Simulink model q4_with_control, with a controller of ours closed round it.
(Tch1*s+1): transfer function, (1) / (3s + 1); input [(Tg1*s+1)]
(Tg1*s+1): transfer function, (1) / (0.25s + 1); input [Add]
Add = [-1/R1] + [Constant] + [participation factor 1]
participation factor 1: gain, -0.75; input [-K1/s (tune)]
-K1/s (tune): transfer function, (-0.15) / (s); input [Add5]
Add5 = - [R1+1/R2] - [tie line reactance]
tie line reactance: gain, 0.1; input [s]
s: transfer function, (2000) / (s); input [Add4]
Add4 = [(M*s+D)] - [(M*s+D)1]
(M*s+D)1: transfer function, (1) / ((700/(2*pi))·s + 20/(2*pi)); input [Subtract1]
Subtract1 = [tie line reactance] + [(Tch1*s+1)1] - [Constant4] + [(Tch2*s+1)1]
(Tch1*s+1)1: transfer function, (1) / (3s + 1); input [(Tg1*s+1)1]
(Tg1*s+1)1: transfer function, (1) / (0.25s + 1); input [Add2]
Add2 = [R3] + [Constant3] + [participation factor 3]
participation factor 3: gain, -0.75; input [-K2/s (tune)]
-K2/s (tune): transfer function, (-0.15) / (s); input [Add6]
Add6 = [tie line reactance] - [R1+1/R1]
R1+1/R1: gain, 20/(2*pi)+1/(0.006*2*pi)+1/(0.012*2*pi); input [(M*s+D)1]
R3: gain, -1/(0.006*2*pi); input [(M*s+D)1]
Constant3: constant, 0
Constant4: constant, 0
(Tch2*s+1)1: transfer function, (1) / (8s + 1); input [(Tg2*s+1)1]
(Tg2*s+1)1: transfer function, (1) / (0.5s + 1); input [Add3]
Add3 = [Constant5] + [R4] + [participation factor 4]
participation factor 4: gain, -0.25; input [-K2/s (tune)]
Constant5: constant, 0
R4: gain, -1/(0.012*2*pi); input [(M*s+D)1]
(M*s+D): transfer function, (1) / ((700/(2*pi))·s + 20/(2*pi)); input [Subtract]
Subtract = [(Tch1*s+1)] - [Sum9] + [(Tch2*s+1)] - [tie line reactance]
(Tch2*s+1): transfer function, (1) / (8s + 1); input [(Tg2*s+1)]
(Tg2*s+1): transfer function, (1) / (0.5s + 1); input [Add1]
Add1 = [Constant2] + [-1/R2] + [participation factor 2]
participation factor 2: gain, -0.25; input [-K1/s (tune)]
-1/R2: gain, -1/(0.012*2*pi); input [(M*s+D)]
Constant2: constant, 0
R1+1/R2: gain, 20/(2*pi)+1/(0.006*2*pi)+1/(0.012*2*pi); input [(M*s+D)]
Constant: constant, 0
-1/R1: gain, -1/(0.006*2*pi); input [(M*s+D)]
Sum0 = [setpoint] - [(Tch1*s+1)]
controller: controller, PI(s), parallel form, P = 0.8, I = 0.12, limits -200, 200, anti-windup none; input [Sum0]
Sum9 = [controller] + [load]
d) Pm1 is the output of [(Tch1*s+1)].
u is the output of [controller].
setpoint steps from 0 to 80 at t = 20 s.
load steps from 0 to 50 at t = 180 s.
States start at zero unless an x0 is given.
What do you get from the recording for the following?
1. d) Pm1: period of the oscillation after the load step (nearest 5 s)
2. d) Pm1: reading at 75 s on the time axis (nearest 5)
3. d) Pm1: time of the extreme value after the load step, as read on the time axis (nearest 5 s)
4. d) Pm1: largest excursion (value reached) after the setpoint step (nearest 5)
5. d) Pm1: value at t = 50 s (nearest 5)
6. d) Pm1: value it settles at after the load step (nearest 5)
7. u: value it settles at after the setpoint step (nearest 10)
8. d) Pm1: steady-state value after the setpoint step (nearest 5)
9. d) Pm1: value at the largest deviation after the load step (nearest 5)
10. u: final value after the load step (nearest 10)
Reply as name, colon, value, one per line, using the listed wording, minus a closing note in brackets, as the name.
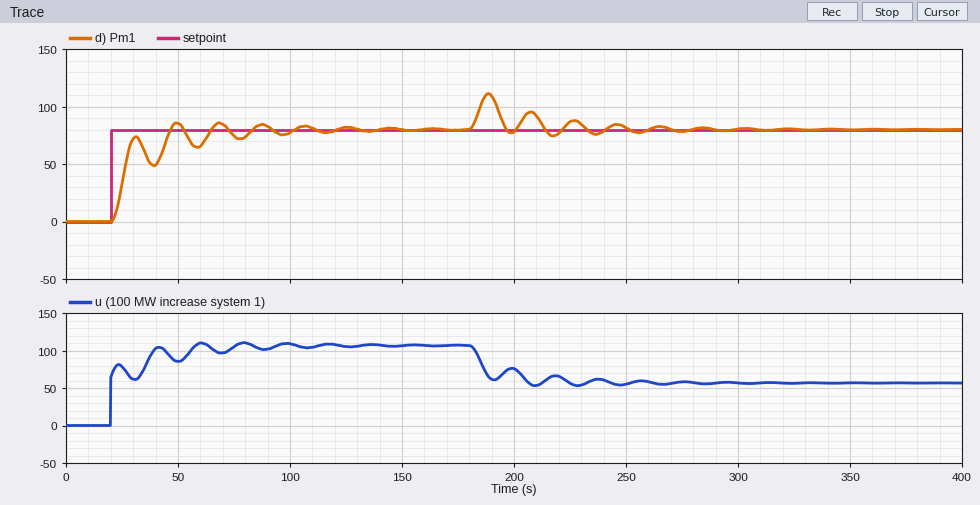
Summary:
d) Pm1: period of the oscillation after the load step: 20 s
d) Pm1: reading at 75 s on the time axis: 75
d) Pm1: time of the extreme value after the load step, as read on the time axis: 190 s
d) Pm1: largest excursion (value reached) after the setpoint step: 85
d) Pm1: value at t = 50 s: 85
d) Pm1: value it settles at after the load step: 80
u: value it settles at after the setpoint step: 110
d) Pm1: steady-state value after the setpoint step: 80
d) Pm1: value at the largest deviation after the load step: 110
u: final value after the load step: 60
